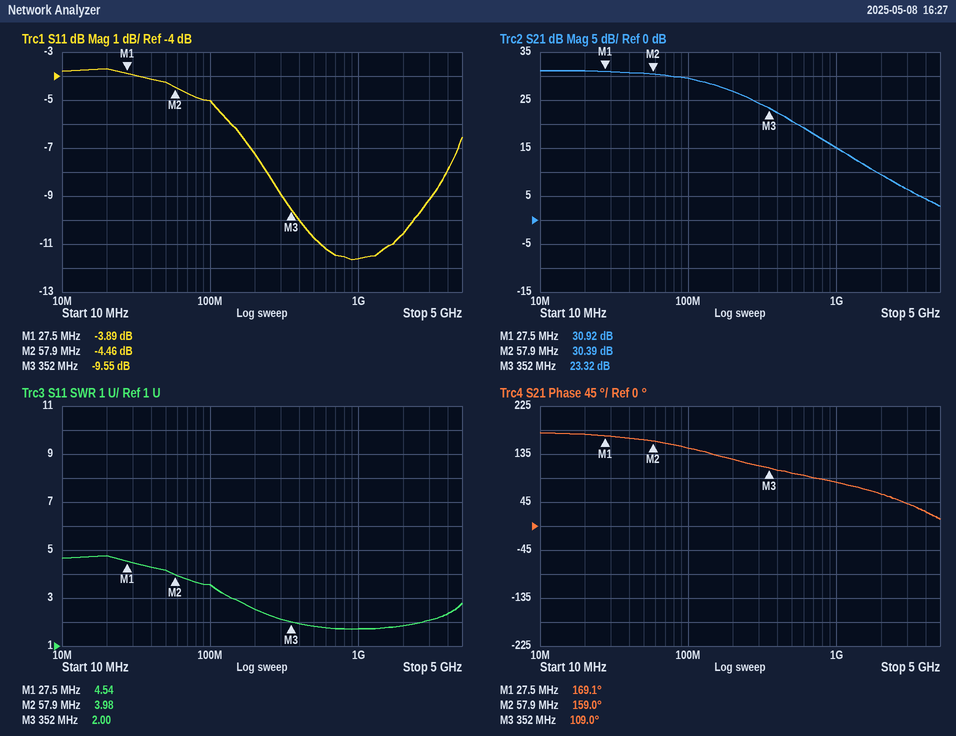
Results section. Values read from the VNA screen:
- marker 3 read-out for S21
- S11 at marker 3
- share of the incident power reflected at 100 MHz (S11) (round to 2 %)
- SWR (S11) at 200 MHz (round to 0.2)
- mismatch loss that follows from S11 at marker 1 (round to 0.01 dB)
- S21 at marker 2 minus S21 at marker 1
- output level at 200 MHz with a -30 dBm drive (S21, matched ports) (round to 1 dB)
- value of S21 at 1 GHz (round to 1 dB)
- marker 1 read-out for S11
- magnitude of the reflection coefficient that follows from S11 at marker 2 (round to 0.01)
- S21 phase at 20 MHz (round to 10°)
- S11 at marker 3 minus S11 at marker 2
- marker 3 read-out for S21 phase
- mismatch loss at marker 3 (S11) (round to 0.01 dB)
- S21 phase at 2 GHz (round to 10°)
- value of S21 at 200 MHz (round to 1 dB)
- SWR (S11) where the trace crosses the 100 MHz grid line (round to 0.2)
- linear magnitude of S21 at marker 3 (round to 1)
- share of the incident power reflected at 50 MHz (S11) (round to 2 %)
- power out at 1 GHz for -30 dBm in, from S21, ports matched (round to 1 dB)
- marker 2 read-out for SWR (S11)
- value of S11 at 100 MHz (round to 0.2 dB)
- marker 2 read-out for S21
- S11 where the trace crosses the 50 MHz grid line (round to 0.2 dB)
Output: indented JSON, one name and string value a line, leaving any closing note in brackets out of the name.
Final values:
{
  "marker 3 read-out for S21": "23.32 dB",
  "S11 at marker 3": "-9.55 dB",
  "share of the incident power reflected at 100 MHz (S11)": "32 %",
  "SWR (S11) at 200 MHz": "2.6",
  "mismatch loss that follows from S11 at marker 1": "2.28 dB",
  "S21 at marker 2 minus S21 at marker 1": "-0.53 dB",
  "output level at 200 MHz with a -30 dBm drive (S21, matched ports)": "-3 dBm",
  "value of S21 at 1 GHz": "15 dB",
  "marker 1 read-out for S11": "-3.89 dB",
  "magnitude of the reflection coefficient that follows from S11 at marker 2": "0.60",
  "S21 phase at 20 MHz": "170°",
  "S11 at marker 3 minus S11 at marker 2": "-5.09 dB",
  "marker 3 read-out for S21 phase": "109.0°",
  "mismatch loss at marker 3 (S11)": "0.51 dB",
  "S21 phase at 2 GHz": "60°",
  "value of S21 at 200 MHz": "27 dB",
  "SWR (S11) where the trace crosses the 100 MHz grid line": "3.6",
  "linear magnitude of S21 at marker 3": "15",
  "share of the incident power reflected at 50 MHz (S11)": "38 %",
  "power out at 1 GHz for -30 dBm in, from S21, ports matched": "-15 dBm",
  "marker 2 read-out for SWR": "3.98",
  "value of S11 at 100 MHz": "-5.0 dB",
  "marker 2 read-out for S21": "30.39 dB",
  "S11 where the trace crosses the 50 MHz grid line": "-4.2 dB"
}
